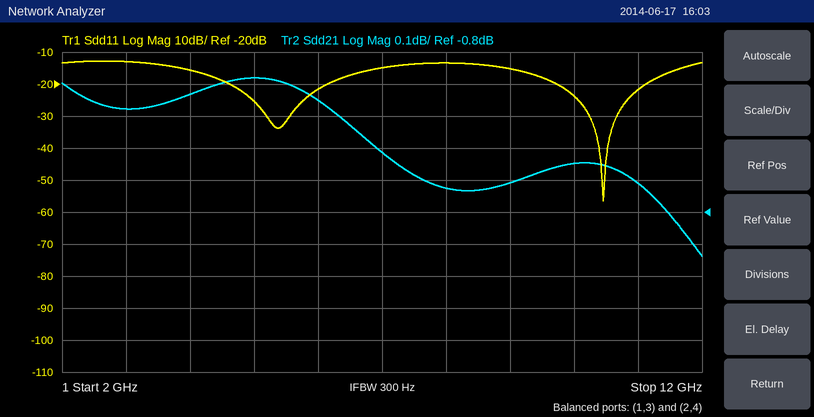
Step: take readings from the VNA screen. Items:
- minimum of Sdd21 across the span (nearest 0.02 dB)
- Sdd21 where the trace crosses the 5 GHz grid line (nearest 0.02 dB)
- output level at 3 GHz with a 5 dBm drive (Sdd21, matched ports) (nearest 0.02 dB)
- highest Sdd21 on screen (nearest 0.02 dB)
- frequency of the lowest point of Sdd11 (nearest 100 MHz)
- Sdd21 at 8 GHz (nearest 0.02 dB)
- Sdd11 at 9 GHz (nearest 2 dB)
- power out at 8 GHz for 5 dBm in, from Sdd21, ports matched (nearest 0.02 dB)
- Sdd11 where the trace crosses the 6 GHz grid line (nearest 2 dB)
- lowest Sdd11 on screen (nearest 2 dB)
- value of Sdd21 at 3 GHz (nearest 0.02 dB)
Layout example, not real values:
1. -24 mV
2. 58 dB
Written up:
1. -0.94 dB
2. -0.38 dB
3. 4.52 dBm
4. -0.38 dB
5. 10.5 GHz
6. -0.72 dB
7. -16 dB
8. 4.28 dBm
9. -22 dB
10. -56 dB
11. -0.48 dB
